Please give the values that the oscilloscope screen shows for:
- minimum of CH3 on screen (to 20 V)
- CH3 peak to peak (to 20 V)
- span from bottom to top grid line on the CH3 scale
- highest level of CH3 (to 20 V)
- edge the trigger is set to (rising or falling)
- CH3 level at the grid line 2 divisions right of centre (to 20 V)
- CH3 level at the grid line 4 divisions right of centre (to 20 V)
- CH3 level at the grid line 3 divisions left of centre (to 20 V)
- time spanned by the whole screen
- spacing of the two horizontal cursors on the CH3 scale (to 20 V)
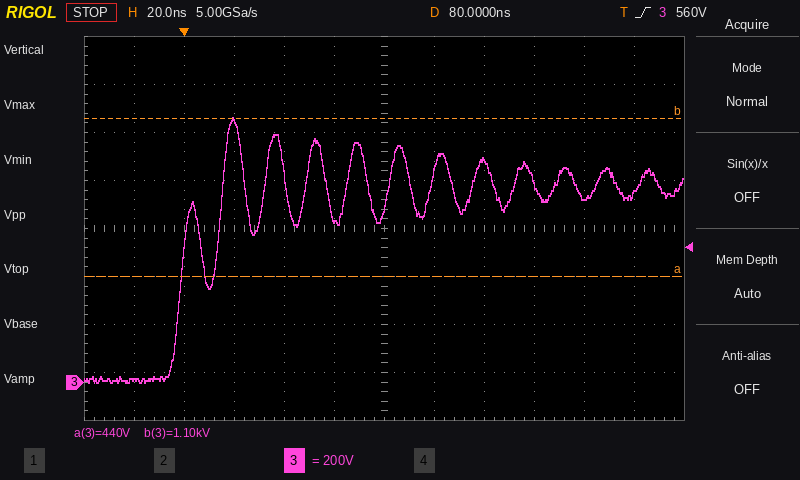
0 V
1.10 kV
1.6 kV
1.10 kV
rising
920 V
760 V
1.08 kV
240 ns
660 V
